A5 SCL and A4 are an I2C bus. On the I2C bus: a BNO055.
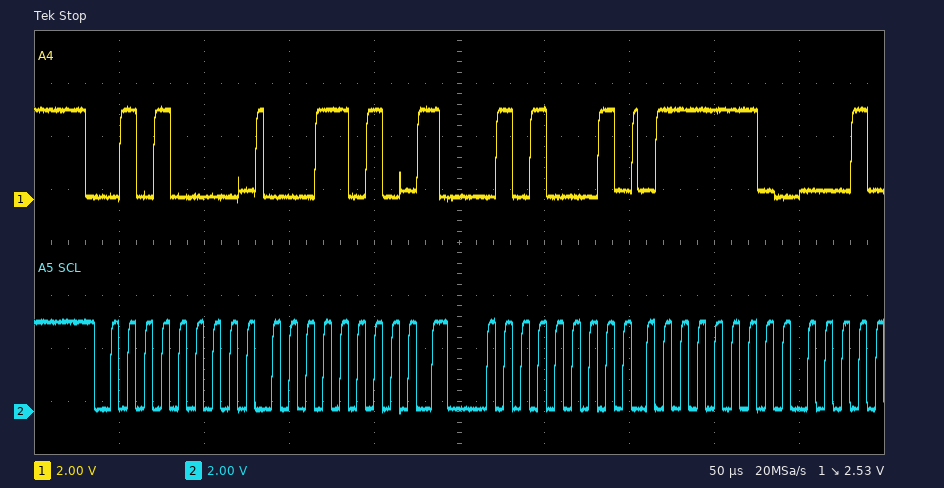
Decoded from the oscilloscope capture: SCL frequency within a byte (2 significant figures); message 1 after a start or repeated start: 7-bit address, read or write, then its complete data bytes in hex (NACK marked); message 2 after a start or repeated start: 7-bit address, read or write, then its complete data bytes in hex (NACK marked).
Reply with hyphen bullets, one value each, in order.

- 100 kHz
- 0x28 write: 1A
- 0x28 read: 7E
